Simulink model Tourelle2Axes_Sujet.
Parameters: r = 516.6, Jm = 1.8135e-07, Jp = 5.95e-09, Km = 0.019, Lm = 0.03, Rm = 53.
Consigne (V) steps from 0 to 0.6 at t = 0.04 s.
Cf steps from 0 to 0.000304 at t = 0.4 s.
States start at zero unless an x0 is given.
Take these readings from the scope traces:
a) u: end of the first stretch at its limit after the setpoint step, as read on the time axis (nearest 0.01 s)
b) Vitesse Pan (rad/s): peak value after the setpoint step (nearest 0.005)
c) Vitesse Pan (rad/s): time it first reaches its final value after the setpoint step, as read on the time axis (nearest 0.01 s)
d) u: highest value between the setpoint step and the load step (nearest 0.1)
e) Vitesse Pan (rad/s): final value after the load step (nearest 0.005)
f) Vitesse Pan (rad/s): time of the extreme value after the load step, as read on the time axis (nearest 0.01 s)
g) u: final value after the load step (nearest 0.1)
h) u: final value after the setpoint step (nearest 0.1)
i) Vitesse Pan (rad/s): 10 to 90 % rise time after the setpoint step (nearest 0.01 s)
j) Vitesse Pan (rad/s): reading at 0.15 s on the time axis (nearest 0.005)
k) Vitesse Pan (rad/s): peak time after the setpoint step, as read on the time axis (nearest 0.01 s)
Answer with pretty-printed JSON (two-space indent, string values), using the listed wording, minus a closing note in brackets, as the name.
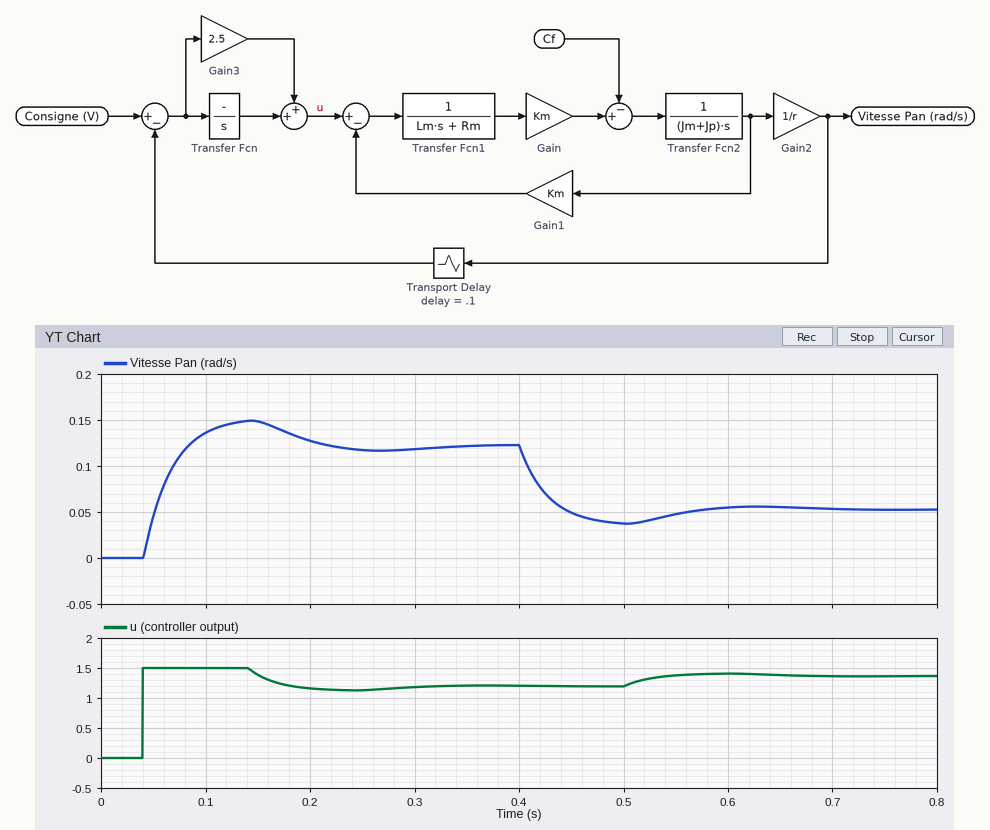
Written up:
{
  "u: end of the first stretch at its limit after the setpoint step, as read on the time axis": "0.14 s",
  "Vitesse Pan (rad/s): peak value after the setpoint step": "0.150",
  "Vitesse Pan (rad/s): time it first reaches its final value after the setpoint step, as read on the time axis": "0.08 s",
  "u: highest value between the setpoint step and the load step": "1.5",
  "Vitesse Pan (rad/s): final value after the load step": "0.055",
  "Vitesse Pan (rad/s): time of the extreme value after the load step, as read on the time axis": "0.50 s",
  "u: final value after the load step": "1.4",
  "u: final value after the setpoint step": "1.2",
  "Vitesse Pan (rad/s): 10 to 90 % rise time after the setpoint step": "0.03 s",
  "Vitesse Pan (rad/s): reading at 0.15 s on the time axis": "0.150",
  "Vitesse Pan (rad/s): peak time after the setpoint step, as read on the time axis": "0.14 s"
}
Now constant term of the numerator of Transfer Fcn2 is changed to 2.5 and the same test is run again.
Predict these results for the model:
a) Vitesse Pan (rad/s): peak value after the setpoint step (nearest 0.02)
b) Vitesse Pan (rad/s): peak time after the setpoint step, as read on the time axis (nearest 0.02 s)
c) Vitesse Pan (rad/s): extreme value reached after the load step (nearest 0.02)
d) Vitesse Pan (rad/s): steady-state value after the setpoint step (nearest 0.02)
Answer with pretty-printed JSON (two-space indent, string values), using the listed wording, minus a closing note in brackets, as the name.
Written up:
{
  "Vitesse Pan (rad/s): peak value after the setpoint step": "0.16",
  "Vitesse Pan (rad/s): peak time after the setpoint step, as read on the time axis": "0.14 s",
  "Vitesse Pan (rad/s): extreme value reached after the load step": "0.04",
  "Vitesse Pan (rad/s): steady-state value after the setpoint step": "0.12"
}
